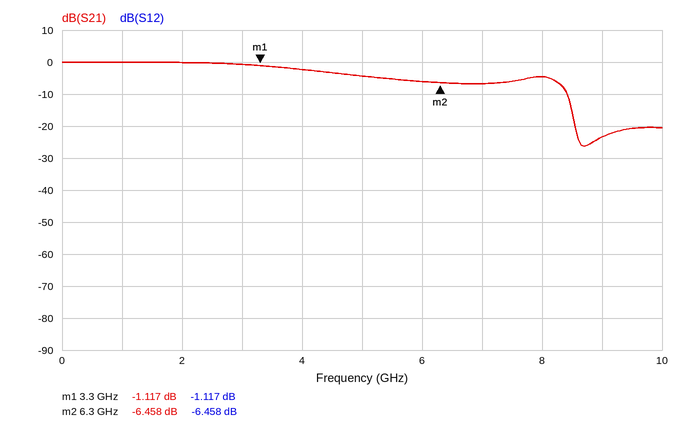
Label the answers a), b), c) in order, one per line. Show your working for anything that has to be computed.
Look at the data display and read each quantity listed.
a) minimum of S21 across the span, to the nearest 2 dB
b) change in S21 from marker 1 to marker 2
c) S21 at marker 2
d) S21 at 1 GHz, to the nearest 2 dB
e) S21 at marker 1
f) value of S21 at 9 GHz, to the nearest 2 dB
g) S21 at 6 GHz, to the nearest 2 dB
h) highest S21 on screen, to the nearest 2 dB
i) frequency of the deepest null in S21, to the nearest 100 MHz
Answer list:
a) -26 dB
b) -6.458 − (-1.117) = -5.341 dB
c) -6.458 dB
d) 0 dB
e) -1.117 dB
f) -24 dB
g) -6 dB
h) 0 dB
i) 8.7 GHz
